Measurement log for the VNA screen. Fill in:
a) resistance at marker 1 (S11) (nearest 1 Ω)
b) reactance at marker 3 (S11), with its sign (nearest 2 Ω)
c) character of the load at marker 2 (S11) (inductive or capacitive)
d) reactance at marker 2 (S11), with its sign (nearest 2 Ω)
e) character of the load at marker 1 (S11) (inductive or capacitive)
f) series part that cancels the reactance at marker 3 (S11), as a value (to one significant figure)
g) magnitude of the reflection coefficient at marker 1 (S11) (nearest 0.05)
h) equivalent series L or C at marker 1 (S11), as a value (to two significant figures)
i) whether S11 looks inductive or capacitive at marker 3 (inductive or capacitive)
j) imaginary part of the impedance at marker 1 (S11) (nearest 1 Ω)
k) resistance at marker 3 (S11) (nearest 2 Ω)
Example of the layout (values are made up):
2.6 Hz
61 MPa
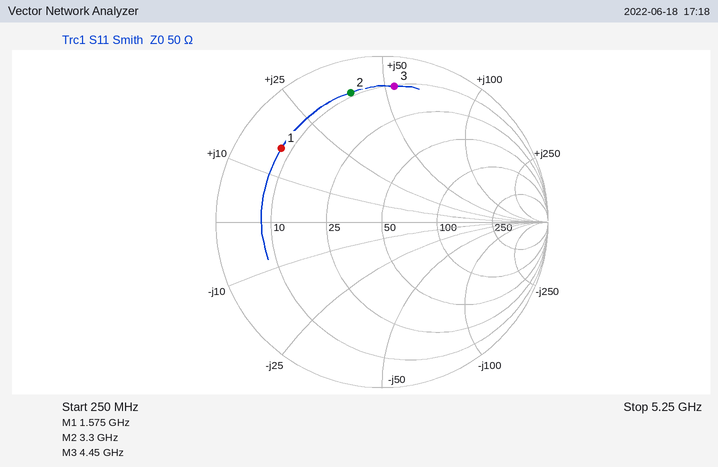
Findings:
8 Ω
+54 Ω
inductive
+38 Ω
inductive
700 fF
0.75
1.6 nH
inductive
+16 Ω
10 Ω
